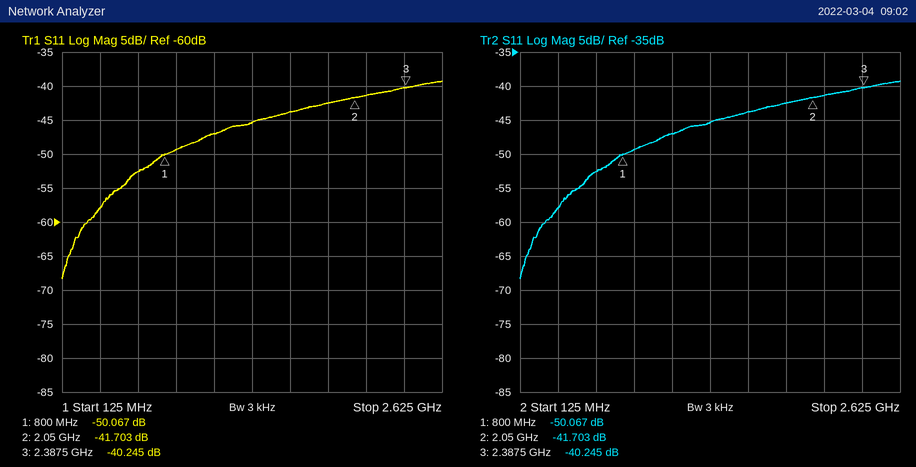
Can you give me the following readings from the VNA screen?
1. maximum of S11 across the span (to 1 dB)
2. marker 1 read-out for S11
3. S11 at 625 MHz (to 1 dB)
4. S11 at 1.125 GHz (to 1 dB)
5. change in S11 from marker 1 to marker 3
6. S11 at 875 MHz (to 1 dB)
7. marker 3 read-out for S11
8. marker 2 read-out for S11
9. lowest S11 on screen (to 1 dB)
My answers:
-39 dB
-50.067 dB
-53 dB
-47 dB
9.822 dB
-49 dB
-40.245 dB
-41.703 dB
-68 dB
